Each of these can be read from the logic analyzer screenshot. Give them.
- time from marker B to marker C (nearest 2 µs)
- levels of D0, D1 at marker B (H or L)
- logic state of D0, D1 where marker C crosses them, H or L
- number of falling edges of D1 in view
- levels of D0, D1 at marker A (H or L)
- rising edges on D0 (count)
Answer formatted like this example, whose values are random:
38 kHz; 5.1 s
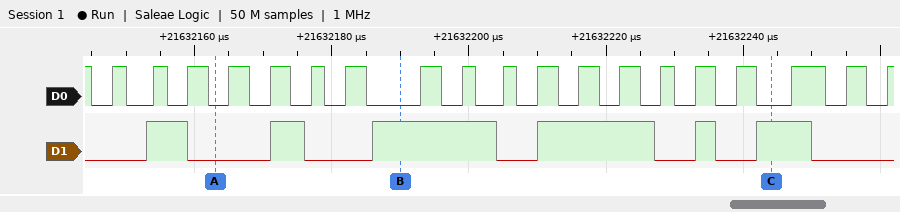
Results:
54 µs; D0=L, D1=H; D0=L, D1=H; 6; D0=L, D1=L; 19
